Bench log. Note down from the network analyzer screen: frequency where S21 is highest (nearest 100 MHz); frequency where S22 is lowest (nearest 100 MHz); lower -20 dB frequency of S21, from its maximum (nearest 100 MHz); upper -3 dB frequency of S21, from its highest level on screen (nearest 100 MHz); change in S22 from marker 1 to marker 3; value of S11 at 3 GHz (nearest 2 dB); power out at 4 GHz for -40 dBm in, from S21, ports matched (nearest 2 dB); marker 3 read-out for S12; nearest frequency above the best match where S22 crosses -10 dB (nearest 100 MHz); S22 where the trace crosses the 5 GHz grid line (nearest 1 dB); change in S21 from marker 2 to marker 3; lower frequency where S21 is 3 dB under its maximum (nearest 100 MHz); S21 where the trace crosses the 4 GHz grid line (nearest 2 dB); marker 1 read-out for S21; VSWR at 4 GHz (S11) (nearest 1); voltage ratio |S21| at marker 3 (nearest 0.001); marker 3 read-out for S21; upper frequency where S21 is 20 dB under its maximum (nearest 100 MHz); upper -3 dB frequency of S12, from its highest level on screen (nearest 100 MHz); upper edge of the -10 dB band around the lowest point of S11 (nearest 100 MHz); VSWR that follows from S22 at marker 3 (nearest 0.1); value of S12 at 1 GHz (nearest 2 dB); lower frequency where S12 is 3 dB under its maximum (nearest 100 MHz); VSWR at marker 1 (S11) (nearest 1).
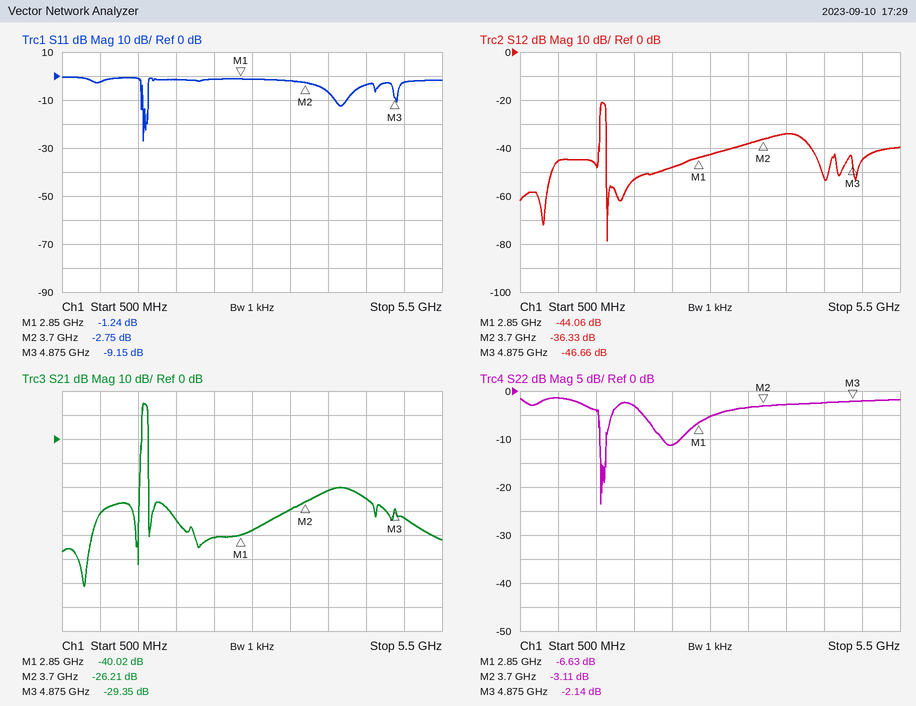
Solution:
1.6 GHz
1.6 GHz
1.5 GHz
1.6 GHz
4.49 dB
-2 dB
-62 dBm
-46.66 dB
1.6 GHz
-2 dB
-3.14 dB
1.6 GHz
-22 dB
-40.02 dB
3
0.034
-29.35 dB
1.6 GHz
1.6 GHz
1.6 GHz
8.2
-46 dB
1.6 GHz
14
